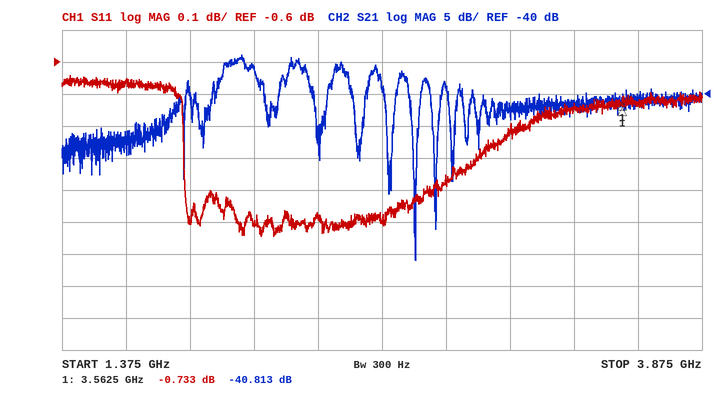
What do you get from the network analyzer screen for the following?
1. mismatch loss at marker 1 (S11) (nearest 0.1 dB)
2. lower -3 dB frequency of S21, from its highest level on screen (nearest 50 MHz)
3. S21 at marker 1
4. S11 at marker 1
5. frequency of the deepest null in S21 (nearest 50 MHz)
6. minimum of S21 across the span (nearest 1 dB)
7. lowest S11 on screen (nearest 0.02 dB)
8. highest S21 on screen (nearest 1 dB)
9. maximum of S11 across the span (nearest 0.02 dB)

8.1 dB
2.00 GHz
-40.813 dB
-0.733 dB
2.75 GHz
-66 dB
-1.14 dB
-34 dB
-0.64 dB
